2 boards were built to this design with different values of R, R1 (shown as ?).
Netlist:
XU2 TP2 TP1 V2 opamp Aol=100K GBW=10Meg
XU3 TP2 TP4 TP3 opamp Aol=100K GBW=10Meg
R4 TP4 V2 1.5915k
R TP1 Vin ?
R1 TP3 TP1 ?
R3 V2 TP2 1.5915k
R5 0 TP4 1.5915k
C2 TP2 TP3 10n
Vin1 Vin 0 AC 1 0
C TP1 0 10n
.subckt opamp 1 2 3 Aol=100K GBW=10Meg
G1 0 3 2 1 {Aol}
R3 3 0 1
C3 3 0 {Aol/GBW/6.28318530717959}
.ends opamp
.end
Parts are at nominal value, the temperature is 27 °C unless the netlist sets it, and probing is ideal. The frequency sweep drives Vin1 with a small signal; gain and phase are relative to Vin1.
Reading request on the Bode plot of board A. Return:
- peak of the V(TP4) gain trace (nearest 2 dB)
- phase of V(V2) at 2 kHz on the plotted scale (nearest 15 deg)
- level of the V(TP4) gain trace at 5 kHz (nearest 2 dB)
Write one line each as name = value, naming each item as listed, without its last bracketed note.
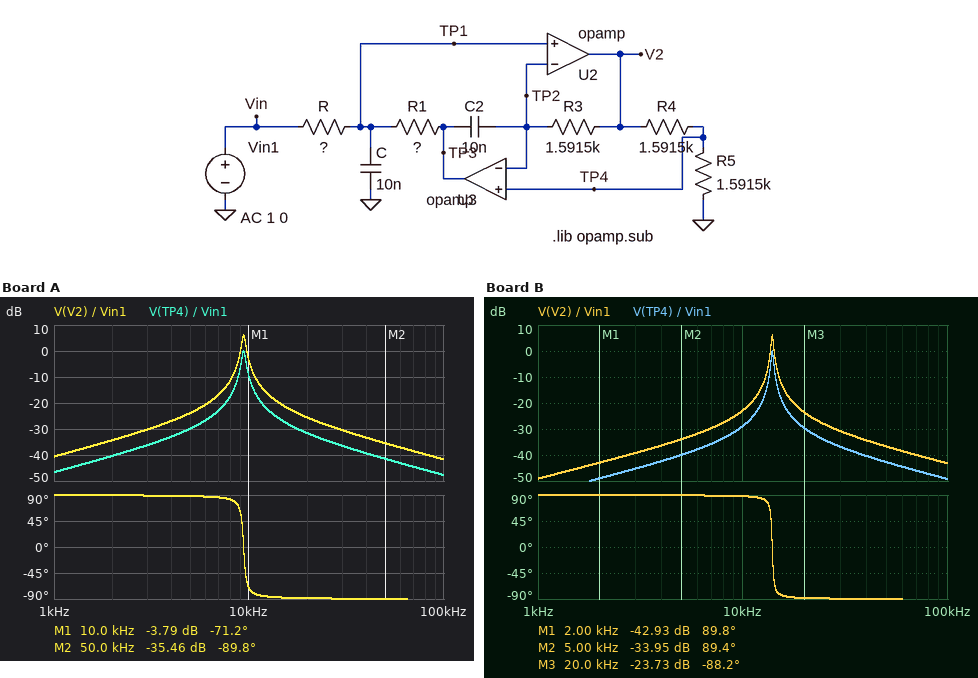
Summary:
peak of the V(TP4) gain trace = 0 dB
phase of V(V2) at 2 kHz on the plotted scale = 90 deg
level of the V(TP4) gain trace at 5 kHz = -30 dB
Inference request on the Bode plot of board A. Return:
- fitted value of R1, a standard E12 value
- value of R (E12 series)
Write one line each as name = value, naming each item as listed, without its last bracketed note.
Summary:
fitted value of R1, a standard E12 value = 1.8 kΩ
value of R = 39 kΩ
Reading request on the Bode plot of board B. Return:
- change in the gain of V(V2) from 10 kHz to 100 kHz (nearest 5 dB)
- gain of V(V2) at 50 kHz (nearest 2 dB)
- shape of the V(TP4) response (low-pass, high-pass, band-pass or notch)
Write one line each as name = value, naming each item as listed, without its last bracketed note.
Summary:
change in the gain of V(V2) from 10 kHz to 100 kHz = -20 dB
gain of V(V2) at 50 kHz = -36 dB
shape of the V(TP4) response = band-pass
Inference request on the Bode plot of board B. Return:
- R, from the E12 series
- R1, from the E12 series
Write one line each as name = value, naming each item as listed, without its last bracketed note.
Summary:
R, from the E12 series = 47 kΩ
R1, from the E12 series = 820 Ω
